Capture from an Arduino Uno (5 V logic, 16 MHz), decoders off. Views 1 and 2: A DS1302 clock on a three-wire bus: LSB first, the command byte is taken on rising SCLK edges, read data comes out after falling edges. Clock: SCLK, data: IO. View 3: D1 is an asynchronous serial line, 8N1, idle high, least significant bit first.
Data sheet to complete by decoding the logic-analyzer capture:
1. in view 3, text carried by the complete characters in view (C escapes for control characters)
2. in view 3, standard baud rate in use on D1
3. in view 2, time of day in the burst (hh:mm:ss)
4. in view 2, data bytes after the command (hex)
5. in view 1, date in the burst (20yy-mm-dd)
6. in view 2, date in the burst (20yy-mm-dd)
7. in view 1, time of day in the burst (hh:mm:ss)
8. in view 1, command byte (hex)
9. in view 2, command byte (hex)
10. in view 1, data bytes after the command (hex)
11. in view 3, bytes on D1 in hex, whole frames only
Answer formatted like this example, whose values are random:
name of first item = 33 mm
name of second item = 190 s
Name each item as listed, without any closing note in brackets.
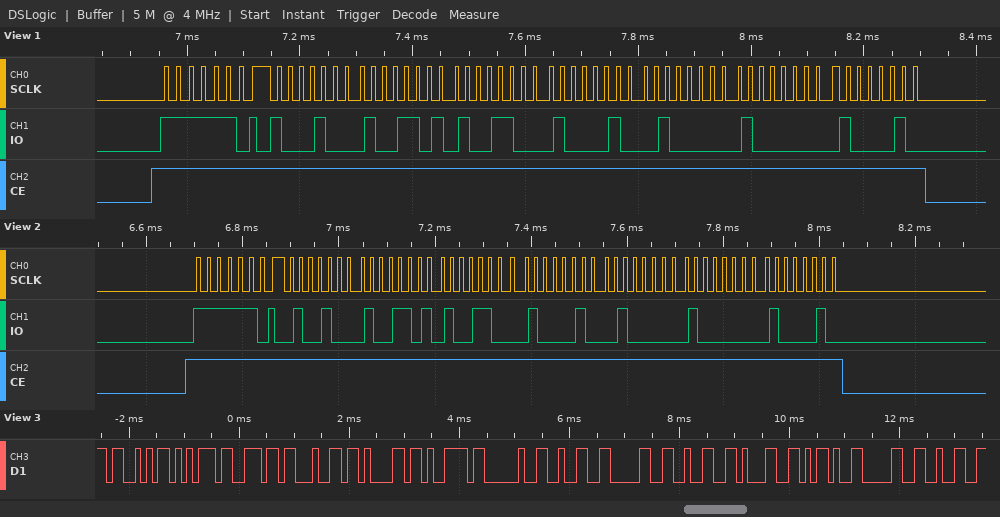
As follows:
in view 3, text carried by the complete characters in view = "Sunday 2021-02"
in view 3, standard baud rate in use on D1 = 9600 baud
in view 2, time of day in the burst = 19:59:12
in view 2, data bytes after the command = 12 59 19 21 02 01 21
in view 1, date in the burst = 2021-02-21
in view 2, date in the burst = 2021-02-21
in view 1, time of day in the burst = 19:59:11
in view 1, command byte = 0xBF
in view 2, command byte = 0xBF
in view 1, data bytes after the command = 11 59 19 21 02 01 21
in view 3, bytes on D1 in hex, whole frames only = 53 75 6E 64 61 79 20 32 30 32 31 2D 30 32
